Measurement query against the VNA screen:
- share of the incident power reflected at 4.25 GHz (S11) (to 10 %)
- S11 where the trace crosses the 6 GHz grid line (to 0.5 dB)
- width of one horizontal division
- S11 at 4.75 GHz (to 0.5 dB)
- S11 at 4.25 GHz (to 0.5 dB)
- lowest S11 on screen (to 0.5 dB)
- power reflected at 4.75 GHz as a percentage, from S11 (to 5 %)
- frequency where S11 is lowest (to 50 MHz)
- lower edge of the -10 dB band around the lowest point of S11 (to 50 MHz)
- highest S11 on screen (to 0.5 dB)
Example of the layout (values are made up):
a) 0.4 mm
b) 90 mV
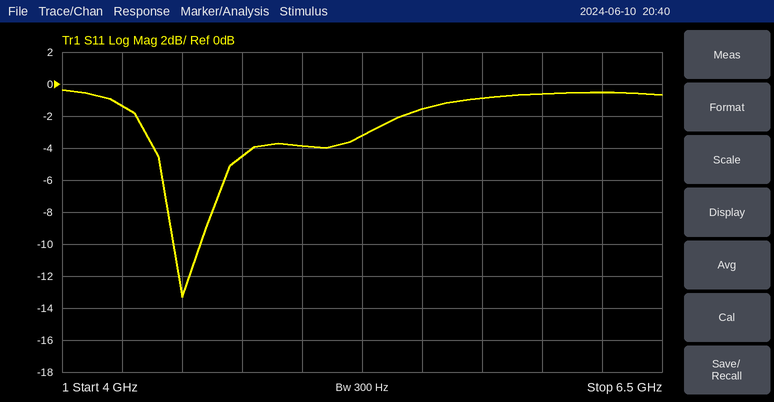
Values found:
a) 70 %
b) -0.5 dB
c) 250 MHz
d) -4.5 dB
e) -1.5 dB
f) -13.5 dB
g) 35 %
h) 4.50 GHz
i) 4.45 GHz
j) -0.5 dB
